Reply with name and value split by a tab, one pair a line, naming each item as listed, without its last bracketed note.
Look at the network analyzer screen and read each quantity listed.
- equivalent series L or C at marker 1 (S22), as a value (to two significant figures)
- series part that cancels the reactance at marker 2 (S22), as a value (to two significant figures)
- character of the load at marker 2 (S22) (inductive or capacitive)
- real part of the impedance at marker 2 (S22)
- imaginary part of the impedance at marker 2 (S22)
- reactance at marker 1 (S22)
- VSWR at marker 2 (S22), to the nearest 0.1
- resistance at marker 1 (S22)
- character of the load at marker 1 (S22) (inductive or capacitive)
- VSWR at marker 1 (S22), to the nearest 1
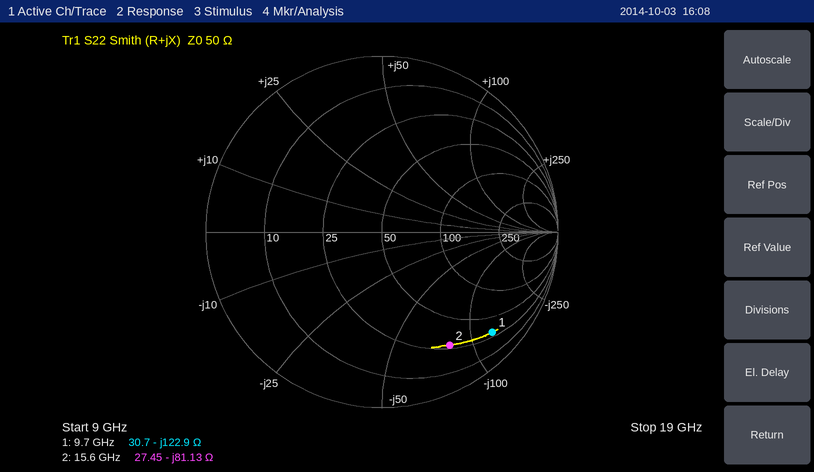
equivalent series L or C at marker 1 (S22), as a value	130 fF
series part that cancels the reactance at marker 2 (S22), as a value	830 pH
character of the load at marker 2 (S22)	capacitive
real part of the impedance at marker 2	27.45 Ω
imaginary part of the impedance at marker 2	-81.13 Ω
reactance at marker 1	-122.9 Ω
VSWR at marker 2 (S22), to the nearest 0.1	7.0
resistance at marker 1	30.7 Ω
character of the load at marker 1 (S22)	capacitive
VSWR at marker 1 (S22), to the nearest 1	12
